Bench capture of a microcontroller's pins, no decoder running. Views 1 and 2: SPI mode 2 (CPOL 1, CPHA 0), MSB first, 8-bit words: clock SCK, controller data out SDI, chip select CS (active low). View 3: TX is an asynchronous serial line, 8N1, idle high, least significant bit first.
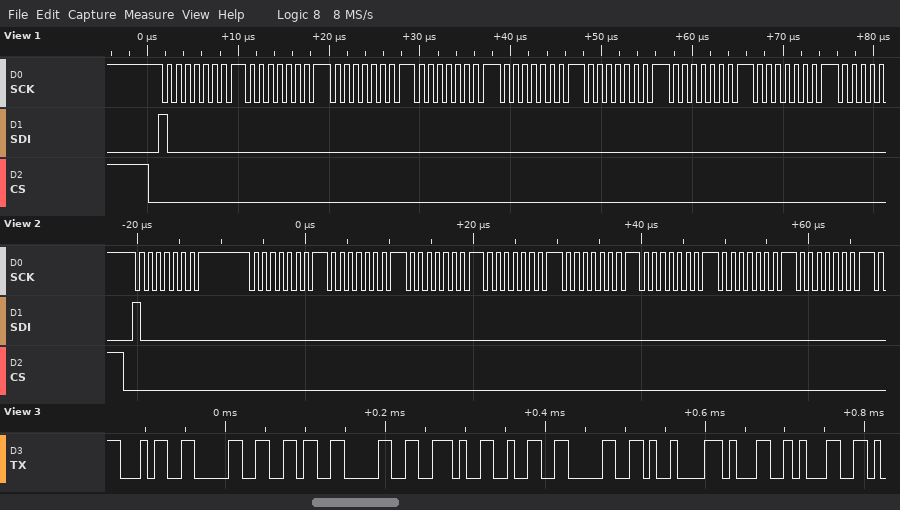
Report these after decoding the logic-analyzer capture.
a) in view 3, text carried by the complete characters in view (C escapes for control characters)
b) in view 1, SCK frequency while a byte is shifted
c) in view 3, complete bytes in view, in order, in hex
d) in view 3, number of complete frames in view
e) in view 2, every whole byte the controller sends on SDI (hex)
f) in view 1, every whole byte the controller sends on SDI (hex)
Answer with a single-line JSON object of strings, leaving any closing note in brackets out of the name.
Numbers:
{"in view 3, text carried by the complete characters in view": "\"4060.20\\t11\"", "in view 1, SCK frequency while a byte is shifted": "1 MHz", "in view 3, complete bytes in view, in order, in hex": "34 30 36 30 2E 32 30 09 31 31", "in view 3, number of complete frames in view": "10", "in view 2, every whole byte the controller sends on SDI": "80 00 00 00 00 00 00 00 00", "in view 1, every whole byte the controller sends on SDI": "0x80 0x00 0x00 0x00 0x00 0x00 0x00 0x00"}
